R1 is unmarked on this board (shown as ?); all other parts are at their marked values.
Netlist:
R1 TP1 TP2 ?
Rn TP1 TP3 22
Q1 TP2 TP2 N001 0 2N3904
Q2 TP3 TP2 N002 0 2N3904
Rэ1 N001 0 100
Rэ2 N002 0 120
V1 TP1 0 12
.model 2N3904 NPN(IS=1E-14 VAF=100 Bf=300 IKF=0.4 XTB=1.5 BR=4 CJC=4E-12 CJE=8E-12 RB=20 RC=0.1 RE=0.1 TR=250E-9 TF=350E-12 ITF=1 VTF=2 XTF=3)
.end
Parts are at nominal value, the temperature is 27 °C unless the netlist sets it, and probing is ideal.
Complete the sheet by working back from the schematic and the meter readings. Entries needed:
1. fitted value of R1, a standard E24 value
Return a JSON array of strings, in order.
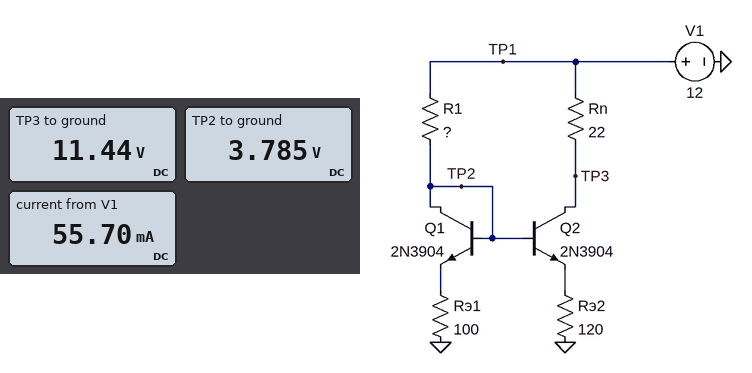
["270 Ω"]
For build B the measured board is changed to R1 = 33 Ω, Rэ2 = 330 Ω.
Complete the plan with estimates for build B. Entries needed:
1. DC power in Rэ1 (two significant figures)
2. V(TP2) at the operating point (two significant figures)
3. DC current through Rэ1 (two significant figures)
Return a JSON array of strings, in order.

["710 mW", "9.2 V", "84 mA"]
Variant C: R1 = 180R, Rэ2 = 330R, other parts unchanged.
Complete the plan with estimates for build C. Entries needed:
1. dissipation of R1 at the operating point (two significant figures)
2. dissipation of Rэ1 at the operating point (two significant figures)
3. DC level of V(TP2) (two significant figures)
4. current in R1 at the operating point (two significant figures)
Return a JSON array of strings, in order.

["290 mW", "160 mW", "4.8 V", "40 mA"]
